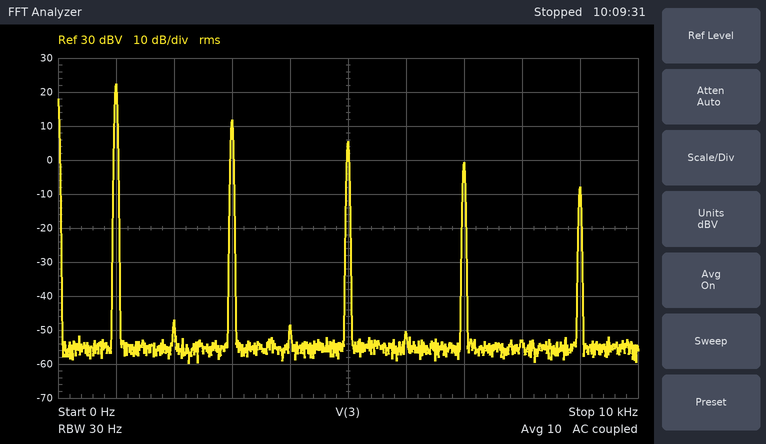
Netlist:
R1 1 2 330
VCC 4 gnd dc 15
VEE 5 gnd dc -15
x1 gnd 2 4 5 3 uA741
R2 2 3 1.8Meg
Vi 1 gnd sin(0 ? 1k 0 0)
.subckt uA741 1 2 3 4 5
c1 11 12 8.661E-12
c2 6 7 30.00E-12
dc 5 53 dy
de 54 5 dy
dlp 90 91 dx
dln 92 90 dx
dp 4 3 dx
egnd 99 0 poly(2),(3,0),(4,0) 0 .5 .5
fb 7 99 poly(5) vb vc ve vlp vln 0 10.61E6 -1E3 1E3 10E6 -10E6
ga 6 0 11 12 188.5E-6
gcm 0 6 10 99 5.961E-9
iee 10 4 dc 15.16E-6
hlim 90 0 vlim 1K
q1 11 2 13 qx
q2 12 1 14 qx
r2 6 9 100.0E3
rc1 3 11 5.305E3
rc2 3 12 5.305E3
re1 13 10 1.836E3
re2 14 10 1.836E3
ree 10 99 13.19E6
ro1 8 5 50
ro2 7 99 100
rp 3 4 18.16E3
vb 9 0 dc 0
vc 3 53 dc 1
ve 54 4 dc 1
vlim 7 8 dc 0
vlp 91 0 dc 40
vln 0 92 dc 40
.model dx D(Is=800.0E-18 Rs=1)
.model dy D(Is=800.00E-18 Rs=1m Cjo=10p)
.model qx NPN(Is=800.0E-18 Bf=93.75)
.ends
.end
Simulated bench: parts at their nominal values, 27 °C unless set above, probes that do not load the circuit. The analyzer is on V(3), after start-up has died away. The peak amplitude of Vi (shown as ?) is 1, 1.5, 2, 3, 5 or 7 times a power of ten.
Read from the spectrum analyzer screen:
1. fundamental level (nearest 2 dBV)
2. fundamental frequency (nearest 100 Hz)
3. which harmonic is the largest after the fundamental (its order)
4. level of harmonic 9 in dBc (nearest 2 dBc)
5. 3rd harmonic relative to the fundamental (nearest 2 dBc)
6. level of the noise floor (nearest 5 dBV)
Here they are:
22 dBV
1.0 kHz
3
-30 dBc
-10 dBc
-55 dBV
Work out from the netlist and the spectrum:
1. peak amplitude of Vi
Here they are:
150 mV
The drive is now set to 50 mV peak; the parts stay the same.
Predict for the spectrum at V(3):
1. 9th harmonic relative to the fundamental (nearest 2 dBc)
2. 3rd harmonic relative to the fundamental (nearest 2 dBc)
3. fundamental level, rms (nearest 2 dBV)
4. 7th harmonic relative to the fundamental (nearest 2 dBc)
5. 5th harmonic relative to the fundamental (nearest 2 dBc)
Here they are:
-34 dBc
-12 dBc
22 dBV
-32 dBc
-24 dBc
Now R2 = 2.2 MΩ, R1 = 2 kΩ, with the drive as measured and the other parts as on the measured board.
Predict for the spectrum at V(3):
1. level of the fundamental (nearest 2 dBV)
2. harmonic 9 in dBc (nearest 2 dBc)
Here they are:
22 dBV
-32 dBc
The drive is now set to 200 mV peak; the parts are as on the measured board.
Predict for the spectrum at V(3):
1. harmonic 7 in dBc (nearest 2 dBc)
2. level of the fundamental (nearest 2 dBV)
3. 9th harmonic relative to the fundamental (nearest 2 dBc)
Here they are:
-22 dBc
22 dBV
-28 dBc
